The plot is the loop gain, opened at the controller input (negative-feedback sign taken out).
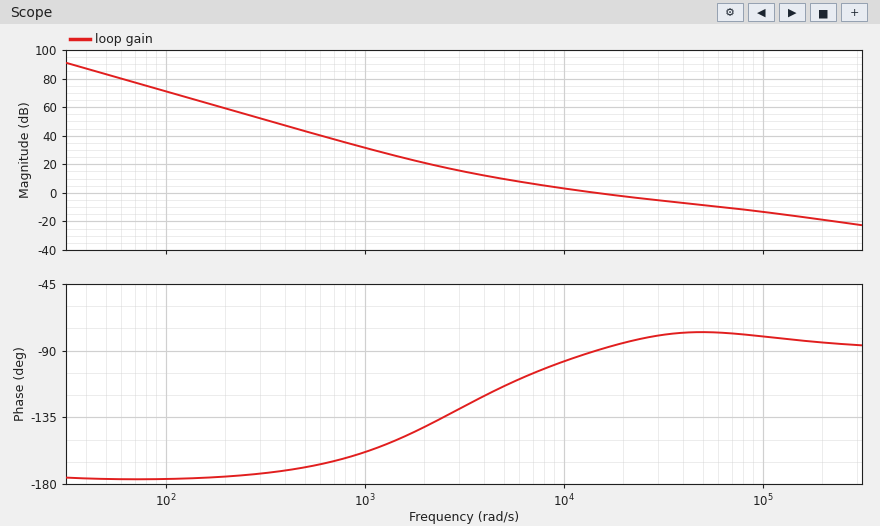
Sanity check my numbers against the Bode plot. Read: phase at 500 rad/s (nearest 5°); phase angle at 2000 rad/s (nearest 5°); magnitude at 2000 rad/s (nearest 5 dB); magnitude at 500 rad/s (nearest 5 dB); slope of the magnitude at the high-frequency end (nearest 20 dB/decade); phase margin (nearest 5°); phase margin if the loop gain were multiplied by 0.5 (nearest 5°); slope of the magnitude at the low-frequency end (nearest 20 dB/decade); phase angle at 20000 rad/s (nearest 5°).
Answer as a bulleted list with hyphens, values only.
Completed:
- -170°
- -140°
- 20 dB
- 45 dB
- -20 dB/decade
- 90°
- 75°
- -40 dB/decade
- -85°
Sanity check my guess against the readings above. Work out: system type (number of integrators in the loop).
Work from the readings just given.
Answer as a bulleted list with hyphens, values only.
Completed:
- 2
